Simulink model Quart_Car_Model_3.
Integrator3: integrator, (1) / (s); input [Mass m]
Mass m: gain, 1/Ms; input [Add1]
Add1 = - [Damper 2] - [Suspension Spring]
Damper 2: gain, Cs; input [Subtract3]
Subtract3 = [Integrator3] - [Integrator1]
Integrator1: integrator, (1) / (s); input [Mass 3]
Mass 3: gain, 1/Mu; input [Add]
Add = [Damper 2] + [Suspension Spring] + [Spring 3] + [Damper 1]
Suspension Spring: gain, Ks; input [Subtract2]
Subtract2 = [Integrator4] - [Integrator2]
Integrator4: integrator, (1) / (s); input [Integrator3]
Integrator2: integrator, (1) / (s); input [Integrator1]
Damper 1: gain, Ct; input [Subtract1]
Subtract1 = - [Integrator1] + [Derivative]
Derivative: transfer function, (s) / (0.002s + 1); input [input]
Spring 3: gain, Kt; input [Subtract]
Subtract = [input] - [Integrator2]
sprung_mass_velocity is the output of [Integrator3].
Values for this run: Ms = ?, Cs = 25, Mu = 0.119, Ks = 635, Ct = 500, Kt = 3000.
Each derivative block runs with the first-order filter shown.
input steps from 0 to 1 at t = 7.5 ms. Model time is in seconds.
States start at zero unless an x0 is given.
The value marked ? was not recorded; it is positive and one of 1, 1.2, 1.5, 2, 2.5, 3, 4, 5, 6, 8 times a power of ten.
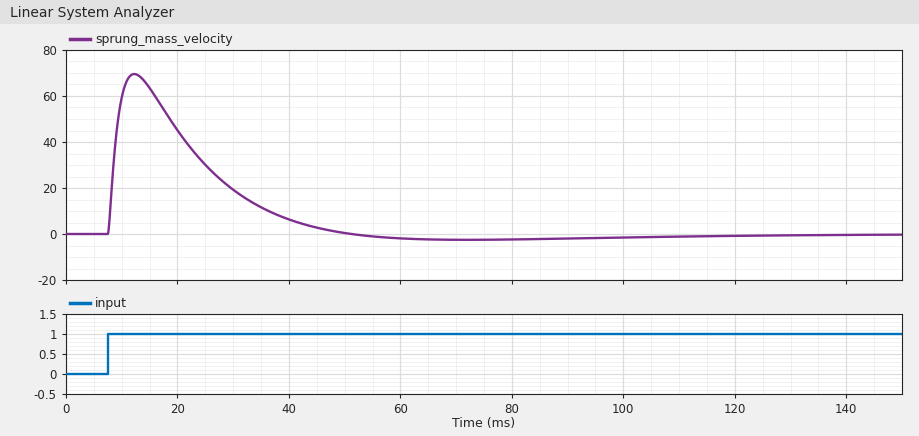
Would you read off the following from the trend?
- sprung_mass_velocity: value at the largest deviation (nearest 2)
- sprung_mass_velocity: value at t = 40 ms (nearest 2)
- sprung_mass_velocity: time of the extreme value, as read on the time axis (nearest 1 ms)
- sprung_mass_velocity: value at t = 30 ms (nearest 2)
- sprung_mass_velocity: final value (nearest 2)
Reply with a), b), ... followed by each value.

a) 70
b) 6
c) 12 ms
d) 20
e) 0
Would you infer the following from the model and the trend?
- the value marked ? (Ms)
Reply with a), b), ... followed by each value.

a) 0.25
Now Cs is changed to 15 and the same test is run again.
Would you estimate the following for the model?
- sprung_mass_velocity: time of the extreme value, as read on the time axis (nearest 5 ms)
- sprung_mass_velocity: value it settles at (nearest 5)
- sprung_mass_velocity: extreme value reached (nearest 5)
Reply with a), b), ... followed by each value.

a) 15 ms
b) 0
c) 50
